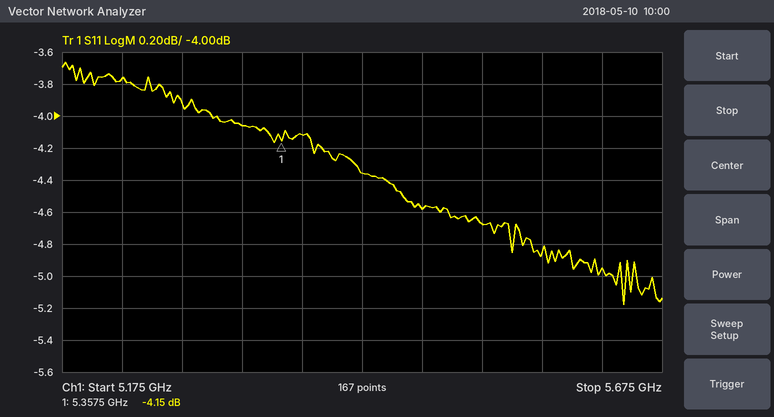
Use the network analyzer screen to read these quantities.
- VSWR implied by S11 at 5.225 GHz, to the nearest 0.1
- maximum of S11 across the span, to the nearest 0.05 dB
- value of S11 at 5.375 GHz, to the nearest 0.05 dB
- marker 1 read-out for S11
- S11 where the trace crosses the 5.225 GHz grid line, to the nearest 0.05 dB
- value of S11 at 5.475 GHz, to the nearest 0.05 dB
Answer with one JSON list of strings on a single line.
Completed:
["4.7", "-3.65 dB", "-4.10 dB", "-4.15 dB", "-3.75 dB", "-4.60 dB"]
